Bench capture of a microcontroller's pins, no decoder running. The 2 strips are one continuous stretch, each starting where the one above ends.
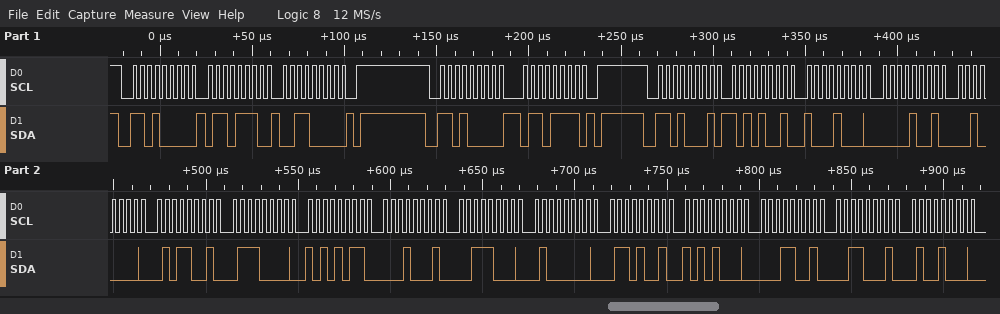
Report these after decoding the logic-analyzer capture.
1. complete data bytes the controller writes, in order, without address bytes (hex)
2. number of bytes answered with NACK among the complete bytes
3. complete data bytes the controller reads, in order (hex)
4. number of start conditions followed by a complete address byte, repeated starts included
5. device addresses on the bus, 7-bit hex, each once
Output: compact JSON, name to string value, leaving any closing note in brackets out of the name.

{"complete data bytes the controller writes, in order, without address bytes": "6E 30 6F", "number of bytes answered with NACK among the complete bytes": "0", "complete data bytes the controller reads, in order": "A9 88 09 20 59 70 AB 11 38 40 69 A8 19 31 48", "number of start conditions followed by a complete address byte, repeated starts included": "3", "device addresses on the bus, 7-bit hex, each once": "0x68"}
